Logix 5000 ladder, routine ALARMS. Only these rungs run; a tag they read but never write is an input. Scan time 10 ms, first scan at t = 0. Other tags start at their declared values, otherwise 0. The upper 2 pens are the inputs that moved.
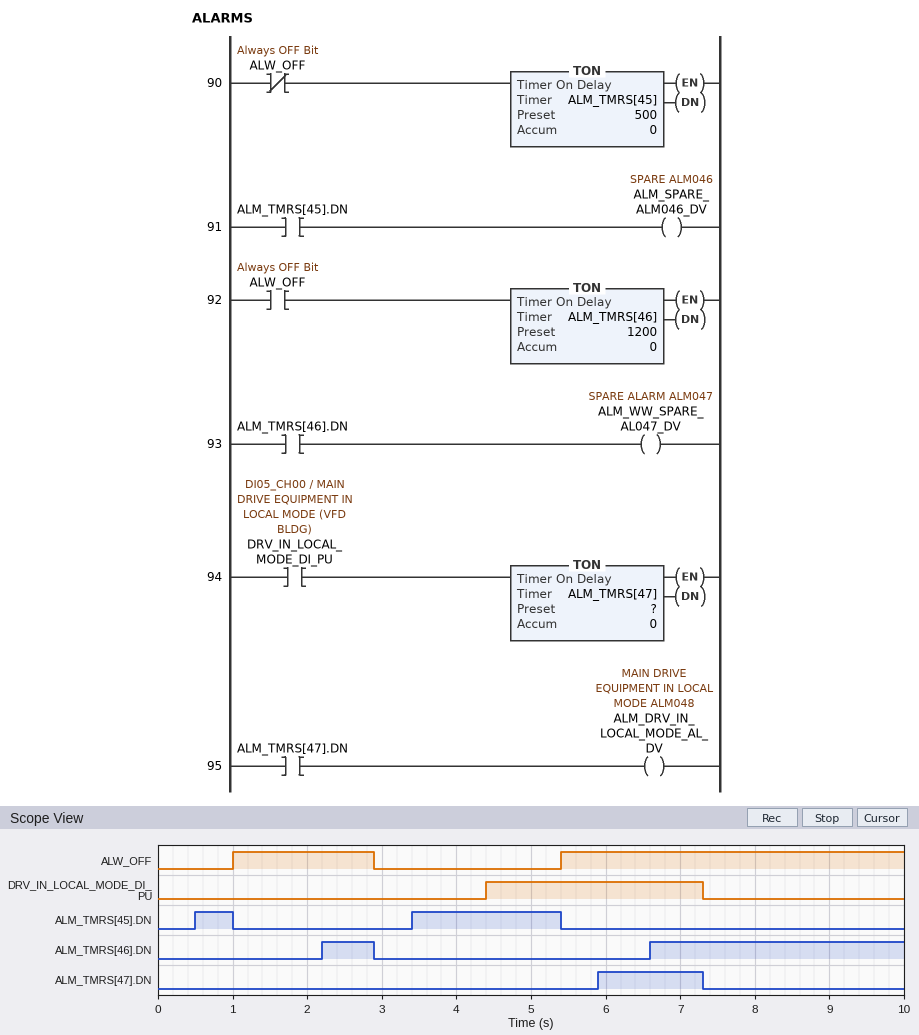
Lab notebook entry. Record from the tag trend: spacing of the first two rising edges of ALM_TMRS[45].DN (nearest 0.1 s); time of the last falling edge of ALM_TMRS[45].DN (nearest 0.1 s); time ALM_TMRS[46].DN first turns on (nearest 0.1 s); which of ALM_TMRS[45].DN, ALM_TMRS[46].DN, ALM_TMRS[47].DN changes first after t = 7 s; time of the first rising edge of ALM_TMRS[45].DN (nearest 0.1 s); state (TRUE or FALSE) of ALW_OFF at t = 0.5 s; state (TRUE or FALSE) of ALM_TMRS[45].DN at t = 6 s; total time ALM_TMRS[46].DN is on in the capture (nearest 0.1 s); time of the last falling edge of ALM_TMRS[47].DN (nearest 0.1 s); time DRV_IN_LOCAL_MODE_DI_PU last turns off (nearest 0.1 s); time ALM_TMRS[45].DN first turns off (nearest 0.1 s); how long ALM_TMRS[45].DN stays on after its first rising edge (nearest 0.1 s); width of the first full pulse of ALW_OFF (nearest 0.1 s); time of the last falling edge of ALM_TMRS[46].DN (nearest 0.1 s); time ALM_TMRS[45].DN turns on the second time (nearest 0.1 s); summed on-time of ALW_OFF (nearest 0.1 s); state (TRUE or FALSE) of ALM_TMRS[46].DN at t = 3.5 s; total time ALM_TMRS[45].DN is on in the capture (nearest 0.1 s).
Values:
2.9 s
5.4 s
2.2 s
ALM_TMRS[47].DN
0.5 s
FALSE
FALSE
4.1 s
7.3 s
7.3 s
1.0 s
0.5 s
1.9 s
2.9 s
3.4 s
6.5 s
FALSE
2.5 s
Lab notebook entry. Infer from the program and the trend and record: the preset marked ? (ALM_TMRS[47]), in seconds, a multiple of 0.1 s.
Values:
1.5 s
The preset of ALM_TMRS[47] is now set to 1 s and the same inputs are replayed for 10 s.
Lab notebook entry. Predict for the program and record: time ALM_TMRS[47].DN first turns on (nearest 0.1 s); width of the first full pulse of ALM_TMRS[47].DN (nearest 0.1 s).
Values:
5.4 s
1.9 s
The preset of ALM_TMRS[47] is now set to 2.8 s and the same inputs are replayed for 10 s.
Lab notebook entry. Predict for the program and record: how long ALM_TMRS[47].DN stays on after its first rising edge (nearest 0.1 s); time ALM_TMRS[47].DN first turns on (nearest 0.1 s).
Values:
0.1 s
7.2 s
